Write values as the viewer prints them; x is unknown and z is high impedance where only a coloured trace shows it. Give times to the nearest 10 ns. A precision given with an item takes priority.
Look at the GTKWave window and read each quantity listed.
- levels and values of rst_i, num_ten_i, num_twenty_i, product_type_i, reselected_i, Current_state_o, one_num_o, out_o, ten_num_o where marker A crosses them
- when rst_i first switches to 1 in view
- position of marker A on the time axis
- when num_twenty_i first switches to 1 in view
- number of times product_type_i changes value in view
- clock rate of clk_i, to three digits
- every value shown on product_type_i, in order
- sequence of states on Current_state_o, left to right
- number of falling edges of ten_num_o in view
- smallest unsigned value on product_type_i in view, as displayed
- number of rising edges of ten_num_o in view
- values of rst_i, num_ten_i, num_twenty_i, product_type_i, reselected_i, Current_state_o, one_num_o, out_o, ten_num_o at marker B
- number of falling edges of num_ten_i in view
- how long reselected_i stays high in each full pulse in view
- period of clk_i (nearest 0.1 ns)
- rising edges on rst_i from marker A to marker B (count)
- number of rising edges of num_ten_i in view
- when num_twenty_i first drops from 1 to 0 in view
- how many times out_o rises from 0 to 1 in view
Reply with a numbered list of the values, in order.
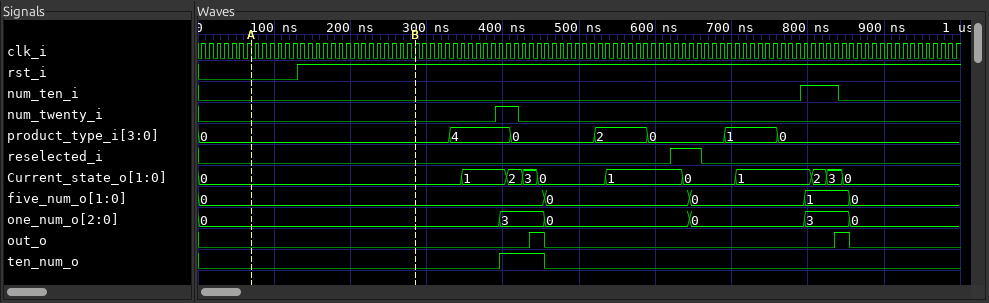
1. rst_i=0, num_ten_i=0, num_twenty_i=0, product_type_i=0, reselected_i=0, Current_state_o=0, one_num_o=0, out_o=0, ten_num_o=0
2. 130 ns
3. 70 ns
4. 390 ns
5. 6
6. 100 MHz
7. 0, 4, 0, 2, 0, 1, 0
8. 0, 1, 2, 3, 0, 1, 0, 1, 2, 3, 0
9. 1
10. 0
11. 1
12. rst_i=1, num_ten_i=0, num_twenty_i=0, product_type_i=0, reselected_i=0, Current_state_o=0, one_num_o=0, out_o=0, ten_num_o=0
13. 1
14. 40 ns
15. 10 ns
16. 1
17. 1
18. 420 ns
19. 2
